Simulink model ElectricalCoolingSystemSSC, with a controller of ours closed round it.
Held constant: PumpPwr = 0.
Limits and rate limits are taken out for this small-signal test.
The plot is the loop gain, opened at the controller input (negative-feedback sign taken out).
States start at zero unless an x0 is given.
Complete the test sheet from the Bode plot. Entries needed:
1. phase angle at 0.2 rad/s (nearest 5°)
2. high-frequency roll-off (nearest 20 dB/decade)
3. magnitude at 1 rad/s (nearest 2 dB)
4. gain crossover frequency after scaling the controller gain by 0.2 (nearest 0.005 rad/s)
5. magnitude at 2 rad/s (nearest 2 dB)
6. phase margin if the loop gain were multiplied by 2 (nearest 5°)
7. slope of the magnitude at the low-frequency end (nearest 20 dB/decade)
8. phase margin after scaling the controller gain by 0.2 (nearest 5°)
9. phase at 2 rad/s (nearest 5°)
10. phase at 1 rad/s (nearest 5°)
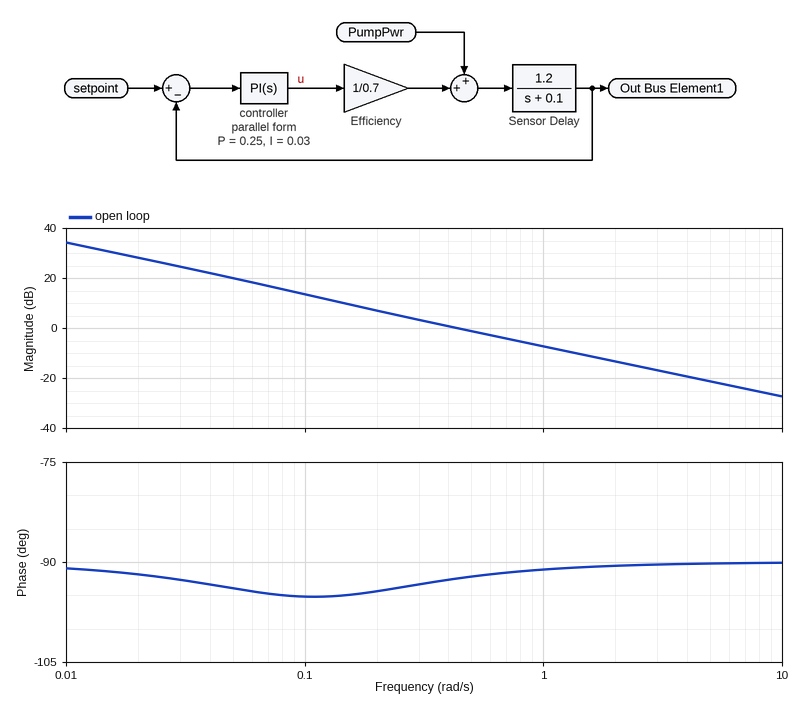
-95°
-20 dB/decade
-8 dB
0.095 rad/s
-14 dB
90°
-20 dB/decade
85°
-90°
-90°
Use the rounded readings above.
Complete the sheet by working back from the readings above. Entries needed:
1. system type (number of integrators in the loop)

1
